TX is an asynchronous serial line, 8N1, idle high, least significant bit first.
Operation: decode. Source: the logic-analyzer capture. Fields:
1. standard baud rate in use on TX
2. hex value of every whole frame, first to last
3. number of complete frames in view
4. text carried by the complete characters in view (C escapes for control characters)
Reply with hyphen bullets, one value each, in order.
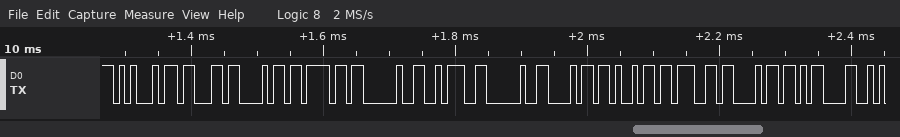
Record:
- 115200 baud
- 45 63 68 6F 20 3A 20 68 69 67 68 0D
- 12
- "Echo : high\r"
